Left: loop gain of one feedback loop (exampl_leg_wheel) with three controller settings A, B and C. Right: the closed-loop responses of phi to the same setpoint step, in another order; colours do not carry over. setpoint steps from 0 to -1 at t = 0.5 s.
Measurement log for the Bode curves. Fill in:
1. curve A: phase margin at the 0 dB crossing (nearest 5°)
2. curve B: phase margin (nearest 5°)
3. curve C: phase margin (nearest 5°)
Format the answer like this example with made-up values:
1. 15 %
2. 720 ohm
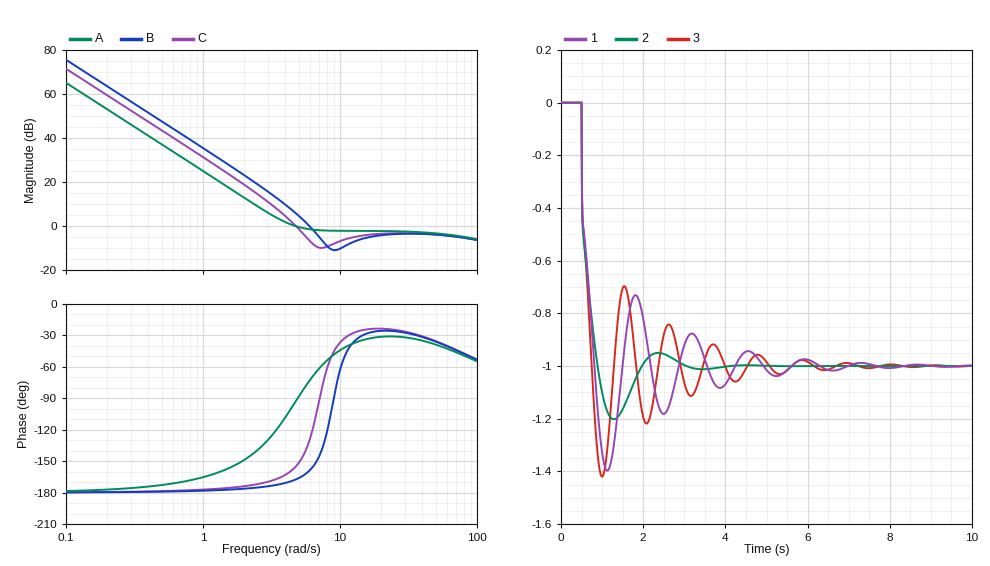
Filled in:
1. 85°
2. 20°
3. 25°
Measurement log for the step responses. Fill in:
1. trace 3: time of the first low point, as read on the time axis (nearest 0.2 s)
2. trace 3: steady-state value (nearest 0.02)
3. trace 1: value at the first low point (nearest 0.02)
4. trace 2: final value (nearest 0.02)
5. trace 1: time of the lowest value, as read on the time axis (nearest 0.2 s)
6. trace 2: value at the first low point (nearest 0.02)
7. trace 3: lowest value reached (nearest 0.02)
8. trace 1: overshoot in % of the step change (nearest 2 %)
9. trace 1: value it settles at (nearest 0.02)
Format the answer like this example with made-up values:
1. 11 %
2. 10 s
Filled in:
1. 1.0 s
2. -1.00
3. -1.40
4. -1.00
5. 1.2 s
6. -1.20
7. -1.42
8. 40 %
9. -1.00
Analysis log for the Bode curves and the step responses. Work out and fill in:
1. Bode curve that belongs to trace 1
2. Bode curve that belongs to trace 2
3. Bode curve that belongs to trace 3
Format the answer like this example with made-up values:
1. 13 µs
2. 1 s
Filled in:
1. C
2. A
3. B
